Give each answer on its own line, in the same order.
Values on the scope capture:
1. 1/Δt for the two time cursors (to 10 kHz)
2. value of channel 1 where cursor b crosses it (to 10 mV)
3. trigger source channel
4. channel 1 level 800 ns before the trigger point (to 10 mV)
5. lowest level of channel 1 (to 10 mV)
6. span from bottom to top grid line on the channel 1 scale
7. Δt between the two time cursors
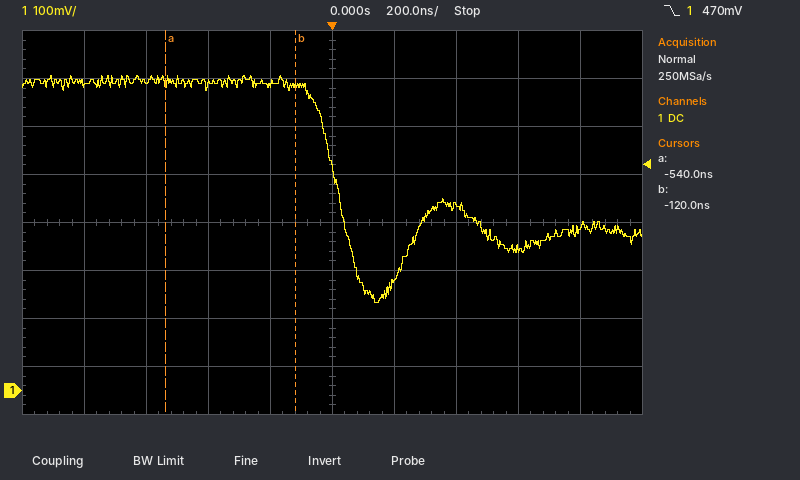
2.38 MHz
640 mV
channel 1
640 mV
180 mV
800 mV
420 ns
